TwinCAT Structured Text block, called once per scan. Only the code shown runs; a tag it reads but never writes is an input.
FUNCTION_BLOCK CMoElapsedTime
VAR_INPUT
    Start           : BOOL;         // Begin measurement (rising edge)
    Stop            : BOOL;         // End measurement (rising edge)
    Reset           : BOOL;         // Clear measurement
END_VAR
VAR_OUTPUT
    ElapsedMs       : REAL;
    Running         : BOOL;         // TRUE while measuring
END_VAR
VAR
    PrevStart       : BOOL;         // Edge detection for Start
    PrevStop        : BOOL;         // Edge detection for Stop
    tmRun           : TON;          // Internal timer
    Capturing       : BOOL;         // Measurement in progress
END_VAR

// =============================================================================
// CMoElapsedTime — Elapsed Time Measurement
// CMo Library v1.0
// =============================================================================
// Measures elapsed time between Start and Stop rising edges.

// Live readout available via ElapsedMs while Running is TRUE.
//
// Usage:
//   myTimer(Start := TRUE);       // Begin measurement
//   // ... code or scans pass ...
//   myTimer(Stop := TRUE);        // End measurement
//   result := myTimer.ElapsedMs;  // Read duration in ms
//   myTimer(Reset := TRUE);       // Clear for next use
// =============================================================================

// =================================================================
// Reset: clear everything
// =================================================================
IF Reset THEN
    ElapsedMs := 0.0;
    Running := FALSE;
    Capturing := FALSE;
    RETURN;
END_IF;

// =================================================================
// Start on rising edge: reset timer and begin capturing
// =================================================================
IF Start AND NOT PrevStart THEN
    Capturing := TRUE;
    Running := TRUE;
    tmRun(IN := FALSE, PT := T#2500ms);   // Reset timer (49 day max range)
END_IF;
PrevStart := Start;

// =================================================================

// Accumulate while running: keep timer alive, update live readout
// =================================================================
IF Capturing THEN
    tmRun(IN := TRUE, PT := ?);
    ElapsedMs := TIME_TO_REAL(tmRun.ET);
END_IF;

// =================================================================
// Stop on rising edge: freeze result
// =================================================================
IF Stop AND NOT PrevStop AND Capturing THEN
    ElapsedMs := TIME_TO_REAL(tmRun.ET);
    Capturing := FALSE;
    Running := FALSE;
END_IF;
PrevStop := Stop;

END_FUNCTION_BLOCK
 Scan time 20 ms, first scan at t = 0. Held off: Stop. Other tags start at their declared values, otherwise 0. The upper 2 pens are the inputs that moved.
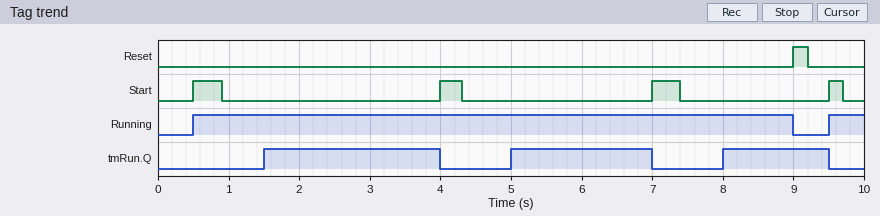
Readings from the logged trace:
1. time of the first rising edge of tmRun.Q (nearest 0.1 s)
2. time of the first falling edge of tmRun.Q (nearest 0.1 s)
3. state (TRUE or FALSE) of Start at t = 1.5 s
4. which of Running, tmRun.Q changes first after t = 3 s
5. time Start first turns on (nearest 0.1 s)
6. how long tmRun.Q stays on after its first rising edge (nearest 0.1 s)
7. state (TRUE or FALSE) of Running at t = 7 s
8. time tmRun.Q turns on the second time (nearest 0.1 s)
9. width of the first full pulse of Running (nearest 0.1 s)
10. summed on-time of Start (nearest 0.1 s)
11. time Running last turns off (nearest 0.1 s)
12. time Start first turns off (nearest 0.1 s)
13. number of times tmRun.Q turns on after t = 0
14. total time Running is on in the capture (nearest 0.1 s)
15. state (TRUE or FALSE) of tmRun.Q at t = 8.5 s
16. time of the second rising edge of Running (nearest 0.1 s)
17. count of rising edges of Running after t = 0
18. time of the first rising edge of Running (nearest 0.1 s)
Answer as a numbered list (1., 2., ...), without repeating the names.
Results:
1. 1.5 s
2. 4.0 s
3. FALSE
4. tmRun.Q
5. 0.5 s
6. 2.5 s
7. TRUE
8. 5.0 s
9. 8.5 s
10. 1.3 s
11. 9.0 s
12. 0.9 s
13. 3
14. 9.0 s
15. TRUE
16. 9.5 s
17. 2
18. 0.5 s
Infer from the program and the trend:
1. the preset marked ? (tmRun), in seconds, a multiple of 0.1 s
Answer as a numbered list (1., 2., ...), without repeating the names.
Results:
1. 1.0 s
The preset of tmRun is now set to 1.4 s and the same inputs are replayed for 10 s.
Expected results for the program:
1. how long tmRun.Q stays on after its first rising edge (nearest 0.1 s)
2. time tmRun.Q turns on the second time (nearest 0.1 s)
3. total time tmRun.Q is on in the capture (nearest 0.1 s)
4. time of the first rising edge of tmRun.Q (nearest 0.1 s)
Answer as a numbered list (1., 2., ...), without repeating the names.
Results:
1. 2.1 s
2. 5.4 s
3. 4.8 s
4. 1.9 s
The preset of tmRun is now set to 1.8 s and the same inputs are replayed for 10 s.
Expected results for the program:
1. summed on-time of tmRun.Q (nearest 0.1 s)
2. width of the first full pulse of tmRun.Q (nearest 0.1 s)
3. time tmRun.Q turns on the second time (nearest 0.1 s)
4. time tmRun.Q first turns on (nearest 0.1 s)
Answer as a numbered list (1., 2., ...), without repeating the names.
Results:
1. 3.6 s
2. 1.7 s
3. 5.8 s
4. 2.3 s
